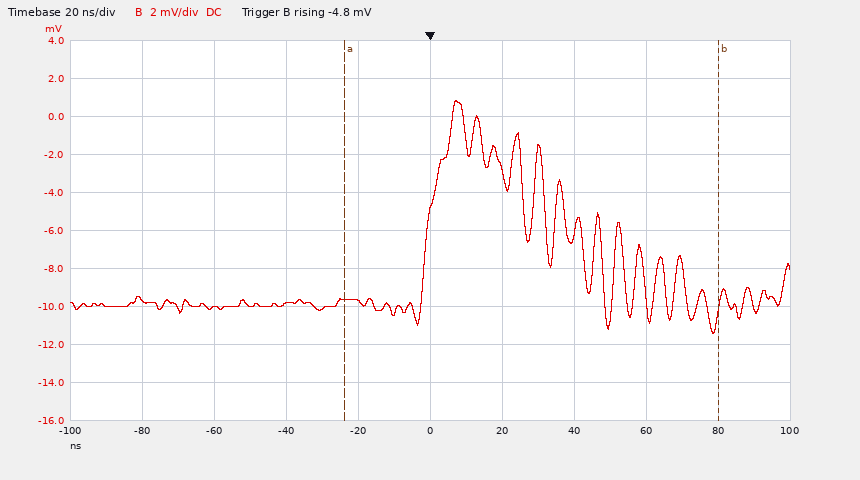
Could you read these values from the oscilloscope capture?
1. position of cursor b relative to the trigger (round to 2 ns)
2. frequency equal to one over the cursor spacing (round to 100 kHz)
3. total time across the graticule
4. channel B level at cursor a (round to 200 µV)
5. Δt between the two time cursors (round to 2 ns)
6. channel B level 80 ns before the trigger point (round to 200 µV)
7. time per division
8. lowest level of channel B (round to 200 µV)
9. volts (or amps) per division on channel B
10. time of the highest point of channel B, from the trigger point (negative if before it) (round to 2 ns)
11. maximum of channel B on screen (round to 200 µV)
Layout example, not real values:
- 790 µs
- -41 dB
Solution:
- +80 ns
- 9.6 MHz
- 200 ns
- -9.6 mV
- 104 ns
- -9.6 mV
- 20 ns
- -11.4 mV
- 2 mV
- +8 ns
- 800 µV
